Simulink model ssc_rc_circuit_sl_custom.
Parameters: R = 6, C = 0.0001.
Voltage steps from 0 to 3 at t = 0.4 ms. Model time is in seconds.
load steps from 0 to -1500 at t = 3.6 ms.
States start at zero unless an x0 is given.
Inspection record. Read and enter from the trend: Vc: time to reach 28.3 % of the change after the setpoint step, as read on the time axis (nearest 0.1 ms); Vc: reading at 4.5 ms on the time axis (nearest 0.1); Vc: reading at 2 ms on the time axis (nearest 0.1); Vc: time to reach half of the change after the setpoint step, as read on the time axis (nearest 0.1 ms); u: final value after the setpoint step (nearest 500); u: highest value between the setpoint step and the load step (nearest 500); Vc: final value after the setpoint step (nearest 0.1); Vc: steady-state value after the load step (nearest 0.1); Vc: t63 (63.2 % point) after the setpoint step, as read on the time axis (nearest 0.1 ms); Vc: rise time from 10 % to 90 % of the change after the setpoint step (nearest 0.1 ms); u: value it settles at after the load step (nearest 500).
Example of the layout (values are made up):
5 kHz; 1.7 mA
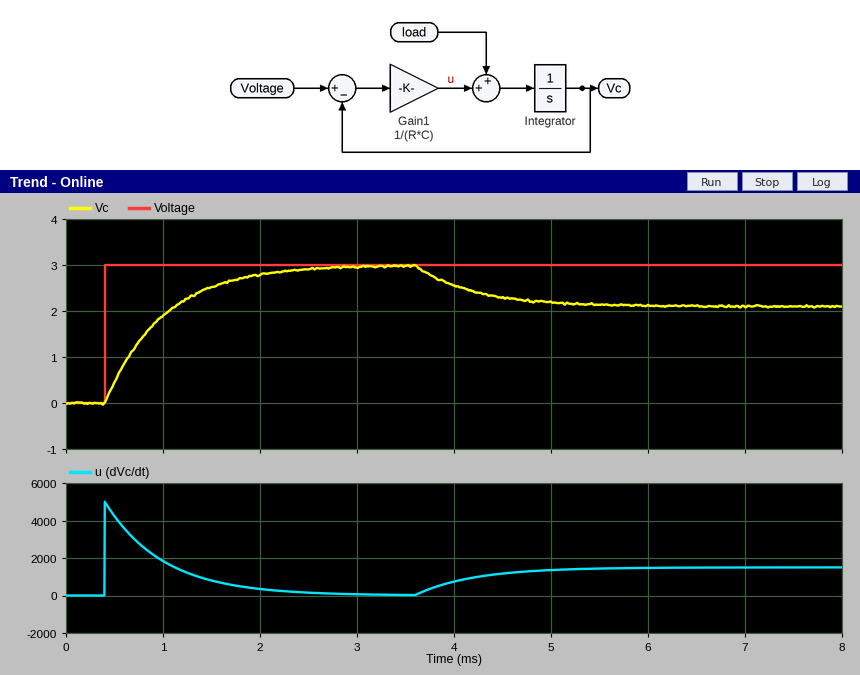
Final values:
0.6 ms; 2.3; 2.8; 0.8 ms; 0; 5000; 3.0; 2.1; 1.0 ms; 1.3 ms; 1500
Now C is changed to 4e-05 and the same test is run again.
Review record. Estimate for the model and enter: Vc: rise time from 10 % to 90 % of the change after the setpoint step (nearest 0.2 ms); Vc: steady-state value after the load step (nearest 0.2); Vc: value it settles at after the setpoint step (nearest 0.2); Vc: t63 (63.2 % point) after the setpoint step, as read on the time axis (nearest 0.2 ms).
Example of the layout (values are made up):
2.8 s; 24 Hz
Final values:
0.6 ms; 2.6; 3.0; 0.6 ms
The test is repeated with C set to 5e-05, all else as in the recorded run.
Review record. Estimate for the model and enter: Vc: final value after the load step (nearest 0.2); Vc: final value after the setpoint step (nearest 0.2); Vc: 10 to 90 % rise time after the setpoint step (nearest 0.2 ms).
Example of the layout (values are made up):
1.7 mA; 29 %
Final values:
2.6; 3.0; 0.6 ms
